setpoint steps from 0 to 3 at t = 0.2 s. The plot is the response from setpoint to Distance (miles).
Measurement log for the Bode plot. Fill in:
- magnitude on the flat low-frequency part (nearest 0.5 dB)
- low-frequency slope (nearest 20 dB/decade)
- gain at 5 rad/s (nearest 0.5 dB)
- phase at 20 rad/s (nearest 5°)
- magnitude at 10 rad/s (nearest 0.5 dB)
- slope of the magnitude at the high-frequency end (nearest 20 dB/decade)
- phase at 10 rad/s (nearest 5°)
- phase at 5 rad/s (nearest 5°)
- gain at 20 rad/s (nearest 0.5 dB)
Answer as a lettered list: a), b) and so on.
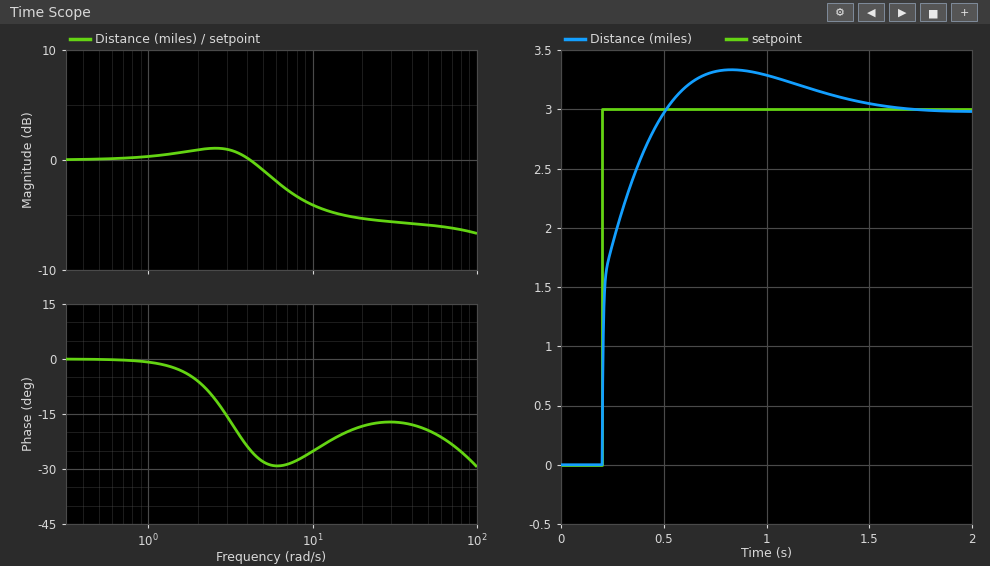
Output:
a) 0.0 dB
b) 0 dB/decade
c) -1.0 dB
d) -20°
e) -4.0 dB
f) 0 dB/decade
g) -25°
h) -30°
i) -5.5 dB
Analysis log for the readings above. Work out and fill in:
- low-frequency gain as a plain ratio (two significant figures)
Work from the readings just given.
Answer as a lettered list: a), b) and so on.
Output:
a) 1.0
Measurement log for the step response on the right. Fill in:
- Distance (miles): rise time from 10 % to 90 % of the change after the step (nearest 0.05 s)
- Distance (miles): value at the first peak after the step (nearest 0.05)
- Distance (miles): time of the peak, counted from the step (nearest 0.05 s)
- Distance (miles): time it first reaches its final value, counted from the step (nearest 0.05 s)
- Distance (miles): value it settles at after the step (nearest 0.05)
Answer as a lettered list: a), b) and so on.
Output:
a) 0.20 s
b) 3.35
c) 0.65 s
d) 0.30 s
e) 3.00
